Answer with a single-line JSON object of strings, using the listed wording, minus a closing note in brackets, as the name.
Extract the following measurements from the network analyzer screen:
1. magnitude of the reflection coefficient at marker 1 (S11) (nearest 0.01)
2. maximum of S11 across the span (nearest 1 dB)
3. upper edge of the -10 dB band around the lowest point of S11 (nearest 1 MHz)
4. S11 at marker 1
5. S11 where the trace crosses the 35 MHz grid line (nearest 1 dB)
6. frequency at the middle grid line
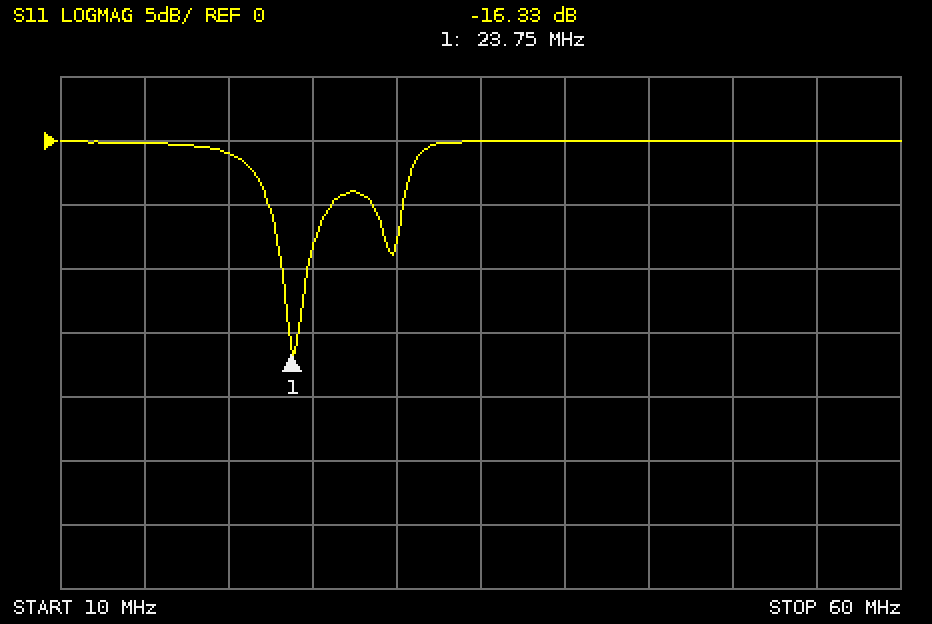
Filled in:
{"magnitude of the reflection coefficient at marker 1 (S11)": "0.15", "maximum of S11 across the span": "0 dB", "upper edge of the -10 dB band around the lowest point of S11": "25 MHz", "S11 at marker 1": "-16.33 dB", "S11 where the trace crosses the 35 MHz grid line": "0 dB", "frequency at the middle grid line": "35 MHz"}
